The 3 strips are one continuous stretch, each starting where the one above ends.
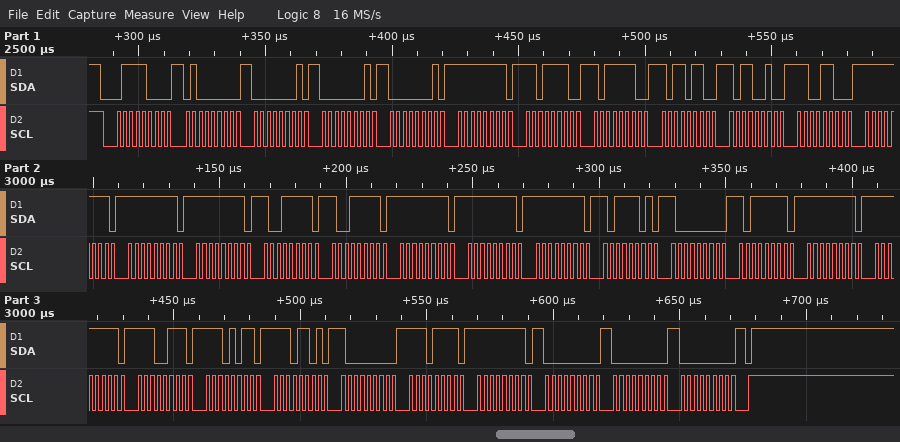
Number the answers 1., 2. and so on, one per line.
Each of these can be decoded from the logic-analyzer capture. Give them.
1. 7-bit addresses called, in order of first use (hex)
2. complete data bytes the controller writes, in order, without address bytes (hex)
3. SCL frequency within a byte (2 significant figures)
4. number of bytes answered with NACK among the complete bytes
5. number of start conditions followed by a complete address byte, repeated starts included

1. 0x3C
2. 40 01 01 01 FF DE BE B6 B2 CC FF FF FF 9F 9F FF FF FF BD 80 BF FF FF E7 EB ED 80 EF FF 00 00 00
3. 400 kHz
4. 0
5. 1
